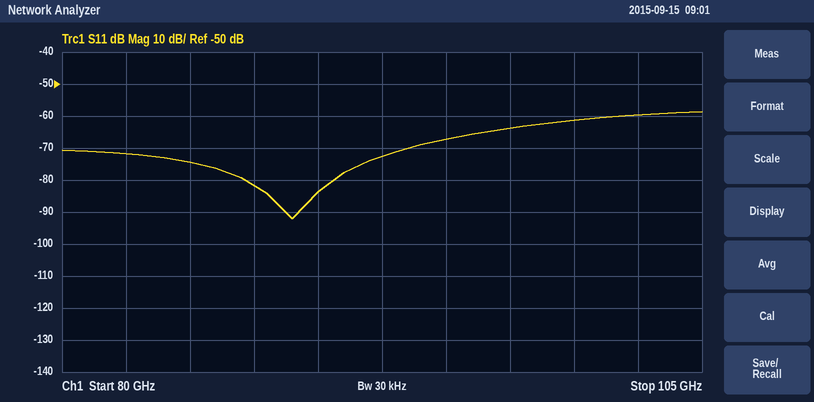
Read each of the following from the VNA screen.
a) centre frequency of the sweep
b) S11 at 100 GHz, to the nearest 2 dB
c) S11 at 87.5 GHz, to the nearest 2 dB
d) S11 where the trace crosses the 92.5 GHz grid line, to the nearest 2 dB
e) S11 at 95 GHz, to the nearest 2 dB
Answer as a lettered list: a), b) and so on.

a) 92.5 GHz
b) -62 dB
c) -82 dB
d) -72 dB
e) -68 dB
